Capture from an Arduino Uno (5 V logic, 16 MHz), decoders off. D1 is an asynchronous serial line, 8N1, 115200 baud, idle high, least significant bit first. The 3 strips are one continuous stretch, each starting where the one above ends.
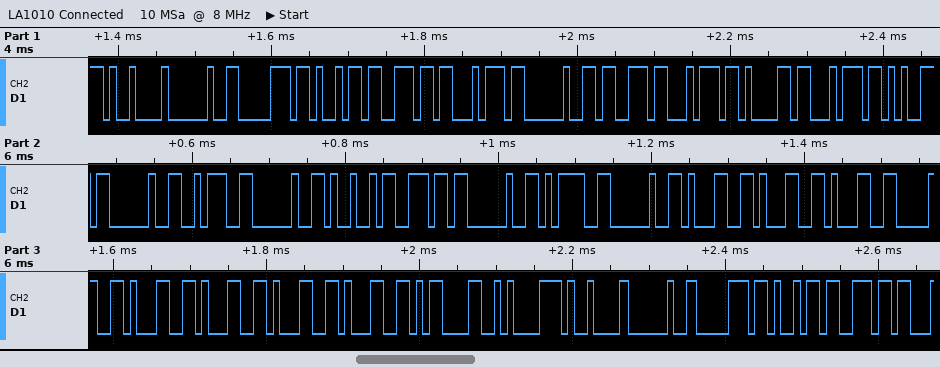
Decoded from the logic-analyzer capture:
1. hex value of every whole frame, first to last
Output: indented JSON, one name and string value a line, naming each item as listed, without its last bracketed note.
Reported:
{
  "hex value of every whole frame, first to last": "09 20 70 69 6E 74 20 73 74 61 74 65 20 3A 20 49 6E 20 3D 20 31 31 31 30 31 31 31 31 0D 0A 09 20 70 69 6E"
}
